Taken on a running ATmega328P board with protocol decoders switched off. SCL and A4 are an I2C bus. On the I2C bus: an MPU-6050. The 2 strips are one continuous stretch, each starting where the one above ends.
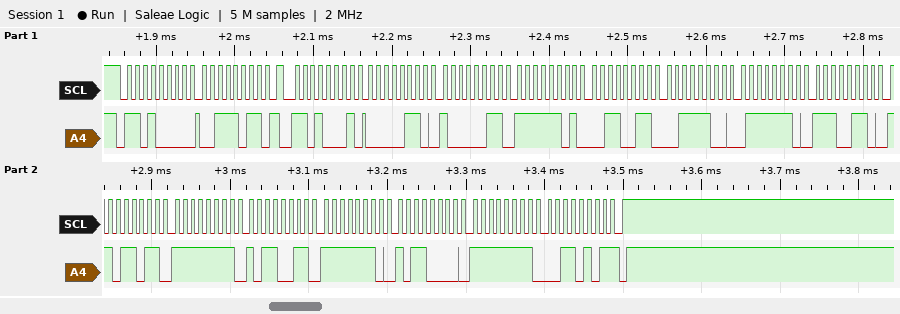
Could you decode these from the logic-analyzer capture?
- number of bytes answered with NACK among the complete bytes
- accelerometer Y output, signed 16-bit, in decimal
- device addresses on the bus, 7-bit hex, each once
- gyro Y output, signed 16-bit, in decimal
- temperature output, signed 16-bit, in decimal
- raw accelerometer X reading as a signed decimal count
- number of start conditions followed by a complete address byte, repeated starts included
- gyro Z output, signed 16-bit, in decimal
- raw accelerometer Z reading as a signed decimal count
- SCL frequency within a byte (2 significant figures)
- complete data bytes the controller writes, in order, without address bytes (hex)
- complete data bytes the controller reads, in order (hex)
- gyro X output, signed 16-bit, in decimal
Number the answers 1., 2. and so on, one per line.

1. 1
2. -717
3. 0x68
4. -336
5. -6437
6. 1667
7. 2
8. -203
9. 15486
10. 100 kHz
11. 3B
12. 06 83 FD 33 3C 7E E6 DB FF B3 FE B0 FF 35
13. -77
